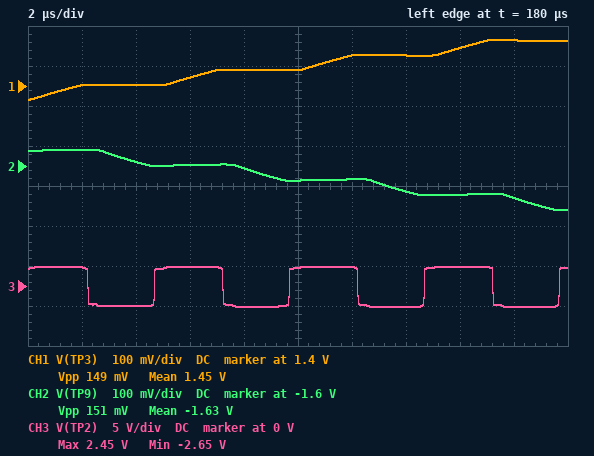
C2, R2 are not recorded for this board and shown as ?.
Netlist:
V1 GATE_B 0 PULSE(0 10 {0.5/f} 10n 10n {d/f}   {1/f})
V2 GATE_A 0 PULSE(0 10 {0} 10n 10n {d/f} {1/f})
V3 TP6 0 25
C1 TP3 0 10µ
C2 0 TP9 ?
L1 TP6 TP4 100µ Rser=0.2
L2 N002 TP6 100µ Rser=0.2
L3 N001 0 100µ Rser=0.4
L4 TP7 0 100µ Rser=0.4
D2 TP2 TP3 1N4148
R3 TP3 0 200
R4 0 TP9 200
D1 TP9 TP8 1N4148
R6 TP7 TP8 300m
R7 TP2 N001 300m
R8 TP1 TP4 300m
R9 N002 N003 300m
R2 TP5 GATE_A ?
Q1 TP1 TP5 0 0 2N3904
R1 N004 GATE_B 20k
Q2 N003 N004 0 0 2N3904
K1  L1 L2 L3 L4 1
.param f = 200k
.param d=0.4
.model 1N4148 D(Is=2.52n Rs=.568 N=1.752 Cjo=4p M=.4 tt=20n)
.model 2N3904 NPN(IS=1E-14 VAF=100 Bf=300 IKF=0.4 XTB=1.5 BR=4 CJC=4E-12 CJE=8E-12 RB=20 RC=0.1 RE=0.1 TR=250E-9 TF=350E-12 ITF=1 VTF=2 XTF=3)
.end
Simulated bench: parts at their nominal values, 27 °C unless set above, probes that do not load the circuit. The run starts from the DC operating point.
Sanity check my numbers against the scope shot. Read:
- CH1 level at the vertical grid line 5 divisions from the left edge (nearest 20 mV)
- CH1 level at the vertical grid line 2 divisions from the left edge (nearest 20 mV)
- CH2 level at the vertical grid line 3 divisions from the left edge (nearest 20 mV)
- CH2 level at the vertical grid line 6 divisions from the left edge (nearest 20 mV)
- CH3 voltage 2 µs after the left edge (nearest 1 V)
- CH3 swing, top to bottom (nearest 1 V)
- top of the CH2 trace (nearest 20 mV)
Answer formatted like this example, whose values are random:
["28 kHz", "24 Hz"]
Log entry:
["1.44 V", "1.40 V", "-1.60 V", "-1.64 V", "2 V", "5 V", "-1.56 V"]
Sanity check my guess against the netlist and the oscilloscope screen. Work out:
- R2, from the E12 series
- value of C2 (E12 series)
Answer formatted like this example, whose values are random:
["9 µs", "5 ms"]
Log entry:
["12 kΩ", "5.6 µF"]
